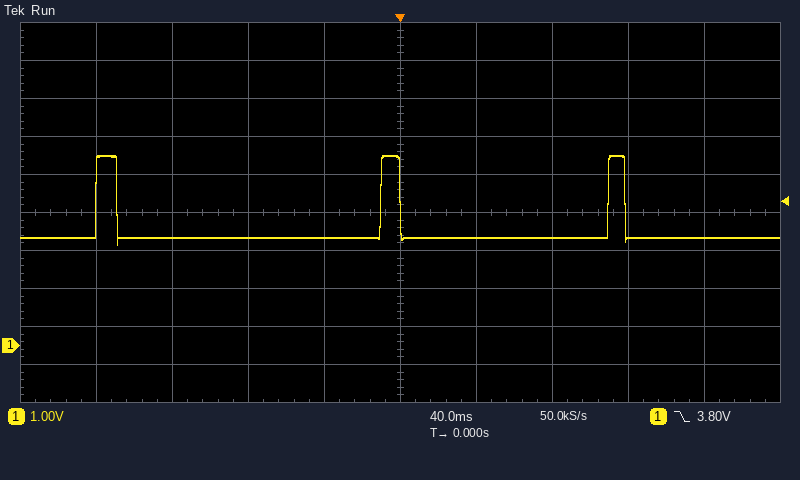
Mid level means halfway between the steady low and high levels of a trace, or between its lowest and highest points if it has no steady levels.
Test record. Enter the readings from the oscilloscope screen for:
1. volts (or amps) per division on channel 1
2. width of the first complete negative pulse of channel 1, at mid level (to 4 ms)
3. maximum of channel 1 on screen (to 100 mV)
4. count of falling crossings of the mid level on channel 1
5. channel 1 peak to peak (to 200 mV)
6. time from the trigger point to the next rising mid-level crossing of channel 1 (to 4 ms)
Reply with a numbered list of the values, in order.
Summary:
1. 1 V
2. 140 ms
3. 5.0 V
4. 3
5. 2.4 V
6. 108 ms
